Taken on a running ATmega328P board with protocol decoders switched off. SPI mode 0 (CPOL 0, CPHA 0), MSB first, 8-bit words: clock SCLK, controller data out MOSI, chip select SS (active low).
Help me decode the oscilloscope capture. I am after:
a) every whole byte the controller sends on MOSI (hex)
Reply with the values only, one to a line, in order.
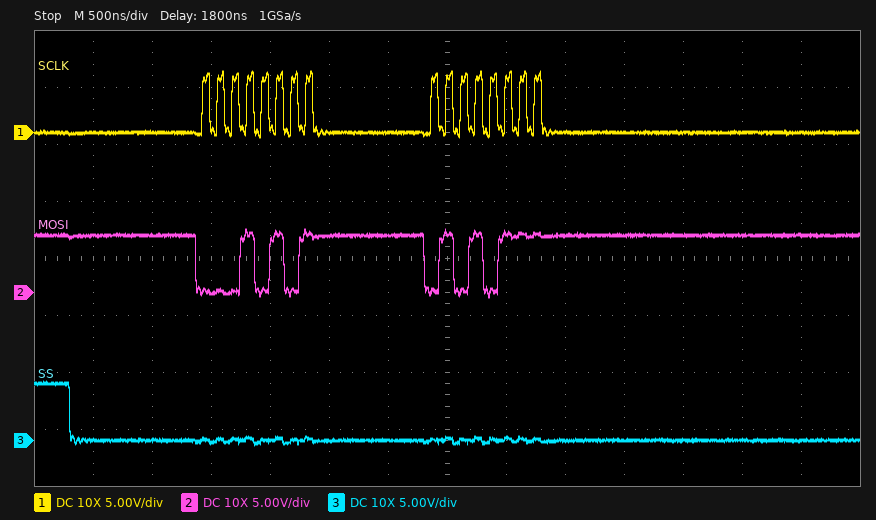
0x15 0x57
